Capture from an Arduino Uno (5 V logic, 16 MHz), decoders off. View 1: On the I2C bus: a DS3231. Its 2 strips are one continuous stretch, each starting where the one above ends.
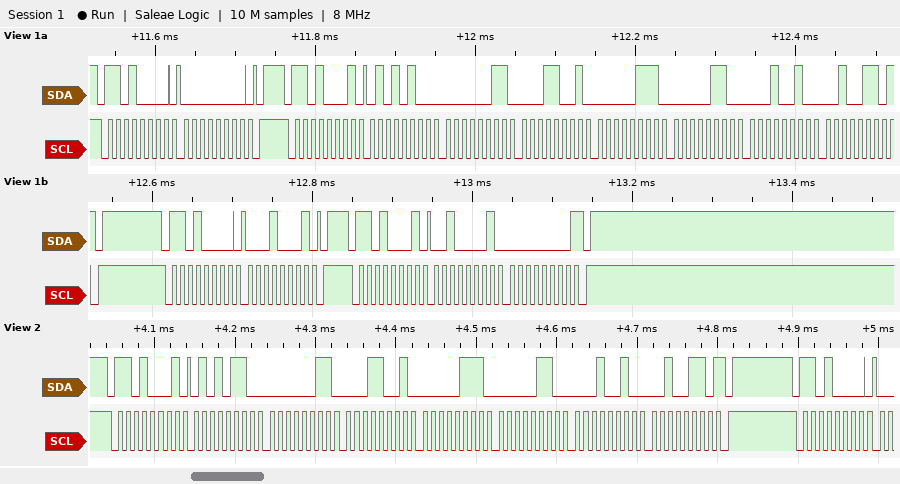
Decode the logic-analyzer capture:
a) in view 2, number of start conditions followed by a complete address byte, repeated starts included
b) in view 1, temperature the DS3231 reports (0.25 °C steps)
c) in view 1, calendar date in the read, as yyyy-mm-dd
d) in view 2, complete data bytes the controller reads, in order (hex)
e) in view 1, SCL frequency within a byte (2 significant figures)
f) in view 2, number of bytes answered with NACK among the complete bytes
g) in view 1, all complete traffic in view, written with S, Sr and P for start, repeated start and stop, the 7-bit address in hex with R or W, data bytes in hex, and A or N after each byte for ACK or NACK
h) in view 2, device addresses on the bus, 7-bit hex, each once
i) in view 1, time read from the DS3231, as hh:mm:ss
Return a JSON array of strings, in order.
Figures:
["2", "33.00 °C", "2026-12-06", "56 03 19 07 06 12 26", "100 kHz", "1", "S 68W A 00 A P S 68R A 54 A 03 A 19 A 07 A 06 A 12 A 26 N P S 68W A 11 A P S 68R A 21 A 00 N P", "0x68", "19:03:54"]
